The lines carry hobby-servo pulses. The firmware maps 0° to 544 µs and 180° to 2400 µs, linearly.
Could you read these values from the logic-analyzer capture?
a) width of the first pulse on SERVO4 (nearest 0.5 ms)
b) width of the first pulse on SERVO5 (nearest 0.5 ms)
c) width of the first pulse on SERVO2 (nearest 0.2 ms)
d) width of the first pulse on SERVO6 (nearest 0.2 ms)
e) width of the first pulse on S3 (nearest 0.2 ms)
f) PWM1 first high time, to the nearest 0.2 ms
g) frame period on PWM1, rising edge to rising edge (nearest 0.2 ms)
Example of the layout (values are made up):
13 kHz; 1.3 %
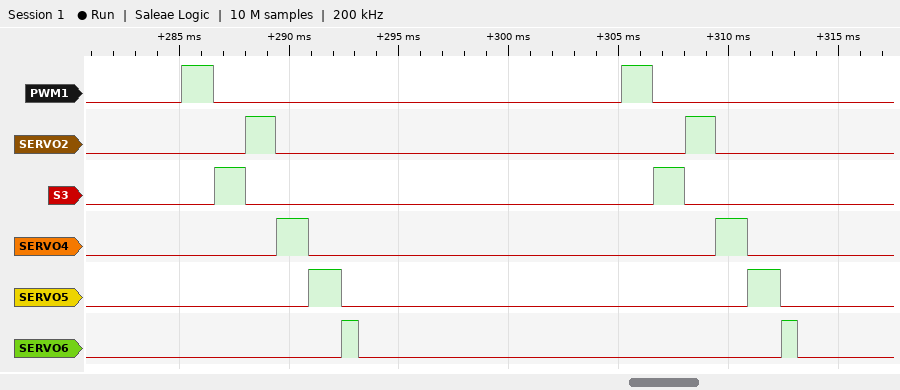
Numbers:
1.5 ms; 1.5 ms; 1.4 ms; 0.8 ms; 1.4 ms; 1.4 ms; 20.0 ms
